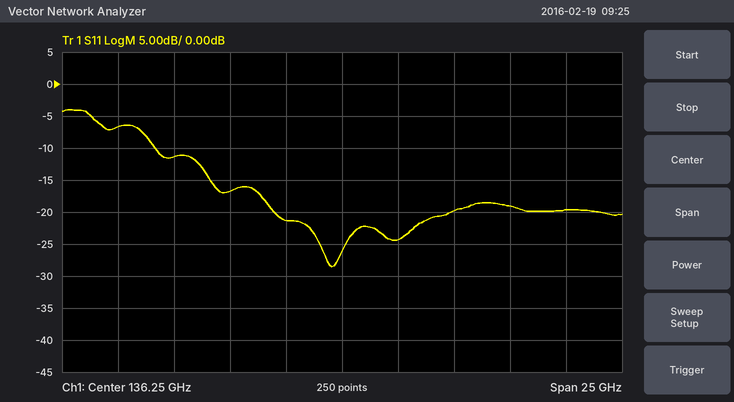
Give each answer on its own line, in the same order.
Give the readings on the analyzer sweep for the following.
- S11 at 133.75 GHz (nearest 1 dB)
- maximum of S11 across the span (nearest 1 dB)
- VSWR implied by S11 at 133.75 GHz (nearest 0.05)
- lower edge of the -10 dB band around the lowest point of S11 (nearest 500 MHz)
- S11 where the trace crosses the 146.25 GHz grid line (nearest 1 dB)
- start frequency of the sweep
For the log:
-21 dB
-4 dB
1.20
128.0 GHz
-20 dB
123.75 GHz
